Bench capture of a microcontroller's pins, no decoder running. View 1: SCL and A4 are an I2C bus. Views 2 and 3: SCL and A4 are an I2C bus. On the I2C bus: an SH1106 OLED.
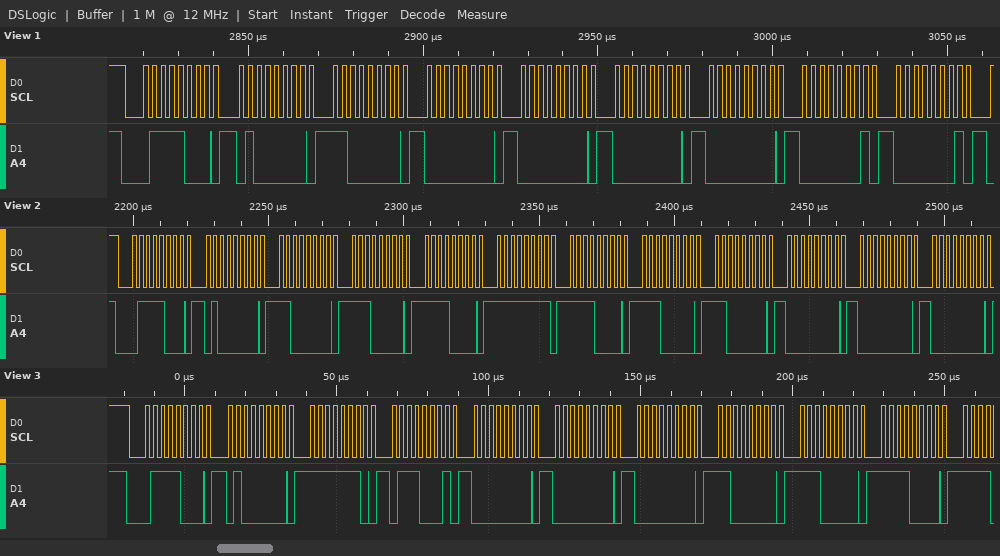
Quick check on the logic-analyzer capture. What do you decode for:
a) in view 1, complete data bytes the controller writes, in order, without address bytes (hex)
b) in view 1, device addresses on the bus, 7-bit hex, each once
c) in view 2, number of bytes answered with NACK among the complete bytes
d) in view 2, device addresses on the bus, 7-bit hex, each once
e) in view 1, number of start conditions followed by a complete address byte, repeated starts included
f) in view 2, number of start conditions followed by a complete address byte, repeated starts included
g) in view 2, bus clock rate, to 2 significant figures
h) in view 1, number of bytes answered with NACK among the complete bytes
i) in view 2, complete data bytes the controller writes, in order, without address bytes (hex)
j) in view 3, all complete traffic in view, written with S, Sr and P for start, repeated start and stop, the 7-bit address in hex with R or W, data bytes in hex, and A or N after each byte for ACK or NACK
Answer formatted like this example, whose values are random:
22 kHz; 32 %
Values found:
40 C0 00 00 00 00 01 01; 0x3C; 0; 0x3C; 1; 1; 400 kHz; 0; 40 C0 E0 F0 FF F0 E0 C0 00 00 00; S 3CW A 40 A FE A 71 A 00 A 00 A 00 A C0 A E0 A F0 A
